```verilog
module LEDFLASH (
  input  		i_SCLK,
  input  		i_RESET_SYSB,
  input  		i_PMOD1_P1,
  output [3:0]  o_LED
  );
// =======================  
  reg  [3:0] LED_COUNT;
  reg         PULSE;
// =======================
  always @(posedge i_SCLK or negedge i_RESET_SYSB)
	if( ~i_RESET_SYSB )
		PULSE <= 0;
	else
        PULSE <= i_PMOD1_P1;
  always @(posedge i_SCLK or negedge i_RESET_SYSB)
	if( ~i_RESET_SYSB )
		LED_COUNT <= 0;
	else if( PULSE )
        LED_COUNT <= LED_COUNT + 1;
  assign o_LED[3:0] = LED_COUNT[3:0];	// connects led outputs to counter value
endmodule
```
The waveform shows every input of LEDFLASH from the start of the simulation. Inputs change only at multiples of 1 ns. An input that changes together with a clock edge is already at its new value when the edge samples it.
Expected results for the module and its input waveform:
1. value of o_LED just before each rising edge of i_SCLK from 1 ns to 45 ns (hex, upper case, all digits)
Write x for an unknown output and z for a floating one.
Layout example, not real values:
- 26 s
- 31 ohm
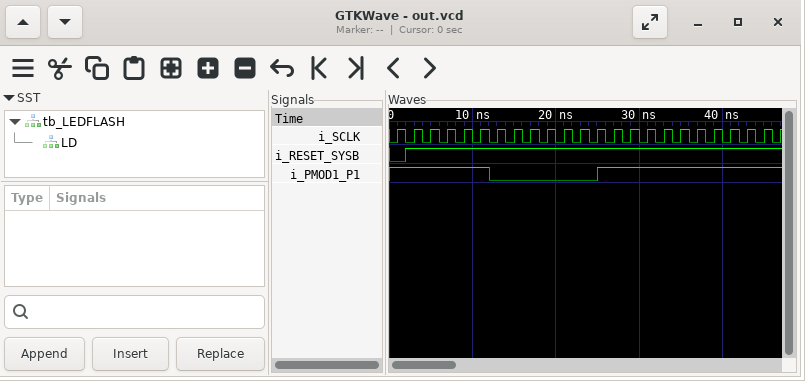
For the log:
- 0, 0, 0, 1, 2, 3, 4, 5, 5, 5, 5, 5, 5, 5, 6, 7, 8, 9, A, B, C, D, E
